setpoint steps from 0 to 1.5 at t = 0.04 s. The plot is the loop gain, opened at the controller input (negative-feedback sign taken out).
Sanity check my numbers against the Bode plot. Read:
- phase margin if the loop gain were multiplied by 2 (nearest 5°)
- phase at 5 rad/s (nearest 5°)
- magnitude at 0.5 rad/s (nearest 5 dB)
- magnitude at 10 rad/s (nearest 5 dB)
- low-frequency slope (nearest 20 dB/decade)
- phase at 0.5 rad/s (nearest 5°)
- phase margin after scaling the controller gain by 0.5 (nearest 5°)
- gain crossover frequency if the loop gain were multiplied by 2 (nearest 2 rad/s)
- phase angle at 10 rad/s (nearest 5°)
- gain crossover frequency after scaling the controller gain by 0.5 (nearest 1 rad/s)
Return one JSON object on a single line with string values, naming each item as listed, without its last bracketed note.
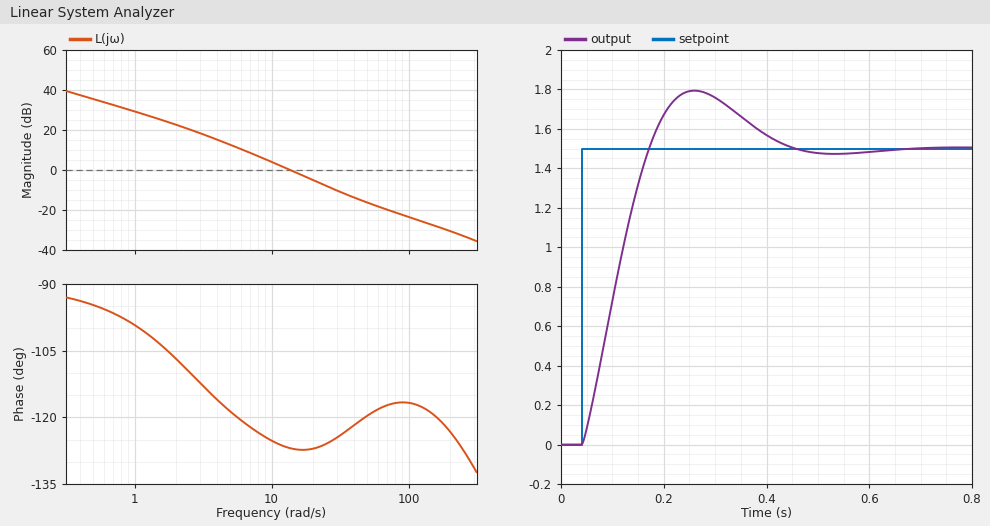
{"phase margin if the loop gain were multiplied by 2": "55°", "phase at 5 rad/s": "-120°", "magnitude at 0.5 rad/s": "35 dB", "magnitude at 10 rad/s": "5 dB", "low-frequency slope": "-20 dB/decade", "phase at 0.5 rad/s": "-95°", "phase margin after scaling the controller gain by 0.5": "55°", "gain crossover frequency if the loop gain were multiplied by 2": "22 rad/s", "phase angle at 10 rad/s": "-125°", "gain crossover frequency after scaling the controller gain by 0.5": "9 rad/s"}
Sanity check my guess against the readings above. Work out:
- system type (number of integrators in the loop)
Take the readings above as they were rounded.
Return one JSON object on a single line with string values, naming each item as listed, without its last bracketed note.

{"system type": "1"}
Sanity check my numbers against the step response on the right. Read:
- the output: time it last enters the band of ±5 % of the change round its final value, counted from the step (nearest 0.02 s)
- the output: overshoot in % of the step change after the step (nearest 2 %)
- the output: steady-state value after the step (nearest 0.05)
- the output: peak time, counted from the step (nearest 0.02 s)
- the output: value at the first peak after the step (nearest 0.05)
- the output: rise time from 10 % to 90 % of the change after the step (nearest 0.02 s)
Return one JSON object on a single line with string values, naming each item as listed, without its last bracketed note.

{"the output: time it last enters the band of ±5 % of the change round its final value, counted from the step": "0.36 s", "the output: overshoot in % of the step change after the step": "20 %", "the output: steady-state value after the step": "1.50", "the output: peak time, counted from the step": "0.22 s", "the output: value at the first peak after the step": "1.80", "the output: rise time from 10 % to 90 % of the change after the step": "0.10 s"}
